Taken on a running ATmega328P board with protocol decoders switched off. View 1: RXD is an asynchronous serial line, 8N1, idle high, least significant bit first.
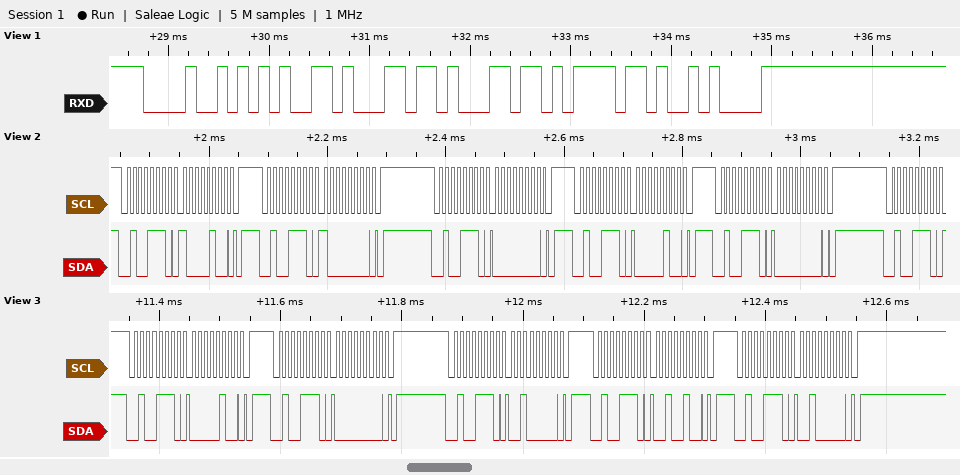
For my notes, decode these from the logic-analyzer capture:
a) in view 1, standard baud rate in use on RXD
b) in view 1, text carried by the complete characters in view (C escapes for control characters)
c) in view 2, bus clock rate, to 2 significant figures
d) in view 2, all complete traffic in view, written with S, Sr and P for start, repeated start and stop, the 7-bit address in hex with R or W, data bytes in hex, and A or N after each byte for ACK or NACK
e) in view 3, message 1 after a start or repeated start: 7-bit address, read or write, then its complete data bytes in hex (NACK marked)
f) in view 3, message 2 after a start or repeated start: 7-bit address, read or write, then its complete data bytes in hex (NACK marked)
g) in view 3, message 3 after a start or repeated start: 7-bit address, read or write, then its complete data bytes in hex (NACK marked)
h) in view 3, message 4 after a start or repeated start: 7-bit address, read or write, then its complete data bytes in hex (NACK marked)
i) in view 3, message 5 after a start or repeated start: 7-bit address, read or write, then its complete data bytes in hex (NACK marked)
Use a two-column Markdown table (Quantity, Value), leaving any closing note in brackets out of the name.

| Quantity | Value |
|---|---|
| in view 1, standard baud rate in use on RXD | 9600 baud |
| in view 1, text carried by the complete characters in view | "Hello\n" |
| in view 2, bus clock rate, to 2 significant figures | 100 kHz |
| in view 2, all complete traffic in view, written with S, Sr and P for start, repeated start and stop, the 7-bit address in hex with R or W, data bytes in hex, and A or N after each byte for ACK or NACK | S 27W A 84 A P S 27W A 80 A P S 27W A 00 A P S 27W A 04 A P S 27W A 00 A P S 27W A |
| in view 3, message 1 after a start or repeated start: 7-bit address, read or write, then its complete data bytes in hex | 0x27 write: 04 |
| in view 3, message 2 after a start or repeated start: 7-bit address, read or write, then its complete data bytes in hex | 0x27 write: 00 |
| in view 3, message 3 after a start or repeated start: 7-bit address, read or write, then its complete data bytes in hex | 0x27 write: 20 |
| in view 3, message 4 after a start or repeated start: 7-bit address, read or write, then its complete data bytes in hex | 0x27 write: 24 |
| in view 3, message 5 after a start or repeated start: 7-bit address, read or write, then its complete data bytes in hex | 0x27 write: 20 |
